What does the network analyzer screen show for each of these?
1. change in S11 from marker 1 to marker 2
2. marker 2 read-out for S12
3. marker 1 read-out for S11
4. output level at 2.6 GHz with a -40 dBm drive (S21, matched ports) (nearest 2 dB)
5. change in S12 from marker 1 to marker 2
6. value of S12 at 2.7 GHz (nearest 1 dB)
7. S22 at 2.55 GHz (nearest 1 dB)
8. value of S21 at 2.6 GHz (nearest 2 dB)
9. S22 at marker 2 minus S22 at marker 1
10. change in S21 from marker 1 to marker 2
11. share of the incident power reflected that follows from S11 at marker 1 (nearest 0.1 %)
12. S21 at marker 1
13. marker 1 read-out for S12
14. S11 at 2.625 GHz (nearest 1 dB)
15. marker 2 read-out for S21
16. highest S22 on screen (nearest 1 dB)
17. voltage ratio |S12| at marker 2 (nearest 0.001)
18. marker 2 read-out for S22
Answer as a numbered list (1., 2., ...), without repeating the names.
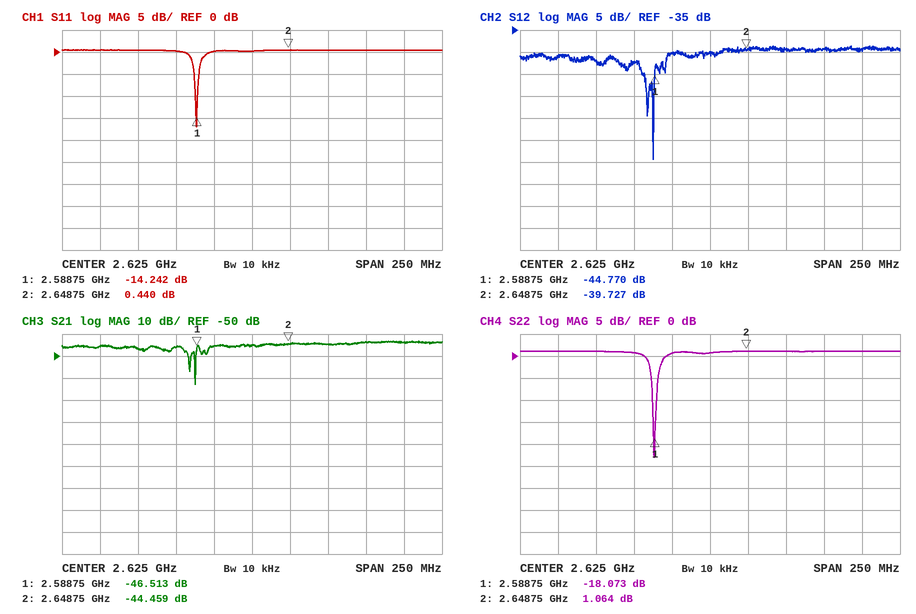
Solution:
1. 14.682 dB
2. -39.727 dB
3. -14.242 dB
4. -86 dBm
5. 5.043 dB
6. -39 dB
7. 1 dB
8. -46 dB
9. 19.137 dB
10. 2.054 dB
11. 3.8 %
12. -46.513 dB
13. -44.770 dB
14. 0 dB
15. -44.459 dB
16. 1 dB
17. 0.010
18. 1.064 dB
